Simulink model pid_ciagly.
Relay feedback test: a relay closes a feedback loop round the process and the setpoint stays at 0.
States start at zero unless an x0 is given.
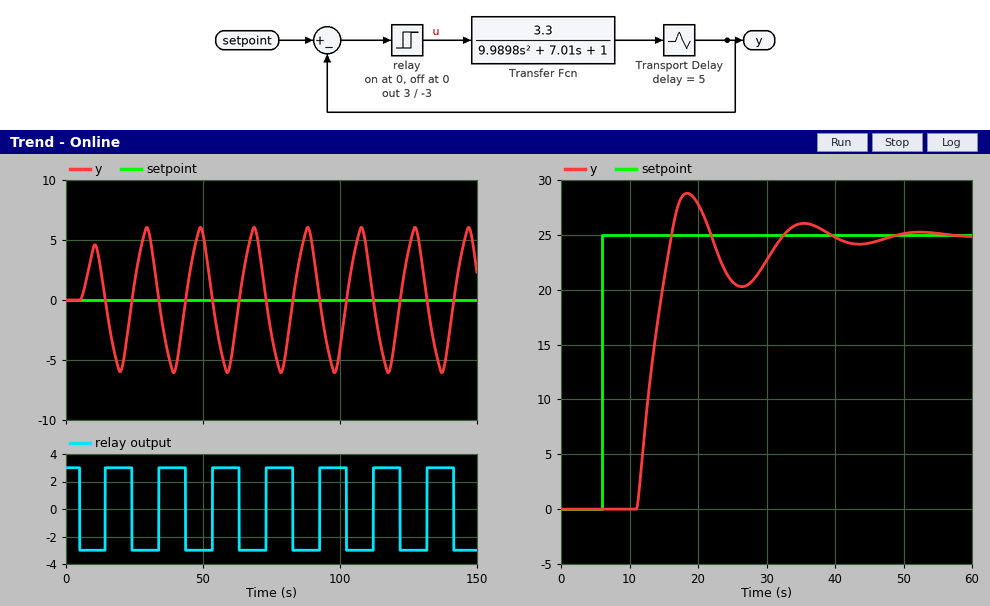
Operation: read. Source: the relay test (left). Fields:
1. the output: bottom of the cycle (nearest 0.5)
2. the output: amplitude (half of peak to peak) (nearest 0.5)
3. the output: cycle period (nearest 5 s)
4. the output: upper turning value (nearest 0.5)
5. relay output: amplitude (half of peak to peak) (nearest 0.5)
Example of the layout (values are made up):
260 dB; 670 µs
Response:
-6.0; 6.0; 20 s; 6.0; 3.0
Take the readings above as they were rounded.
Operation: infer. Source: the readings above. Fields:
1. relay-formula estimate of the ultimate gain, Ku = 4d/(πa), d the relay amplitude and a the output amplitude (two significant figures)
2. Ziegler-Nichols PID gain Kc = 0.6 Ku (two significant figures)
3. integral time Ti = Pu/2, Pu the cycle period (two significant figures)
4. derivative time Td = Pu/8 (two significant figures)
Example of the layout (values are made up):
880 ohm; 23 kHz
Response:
0.64; 0.38; 10 s; 2.5 s
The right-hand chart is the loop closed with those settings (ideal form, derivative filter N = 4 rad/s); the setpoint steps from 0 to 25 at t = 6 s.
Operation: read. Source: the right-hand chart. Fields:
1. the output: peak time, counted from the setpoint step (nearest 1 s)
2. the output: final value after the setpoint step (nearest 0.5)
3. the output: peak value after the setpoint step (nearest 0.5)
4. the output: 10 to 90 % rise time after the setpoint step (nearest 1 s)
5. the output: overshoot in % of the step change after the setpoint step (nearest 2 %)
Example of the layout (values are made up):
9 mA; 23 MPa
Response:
12 s; 25.0; 29.0; 4 s; 16 %
